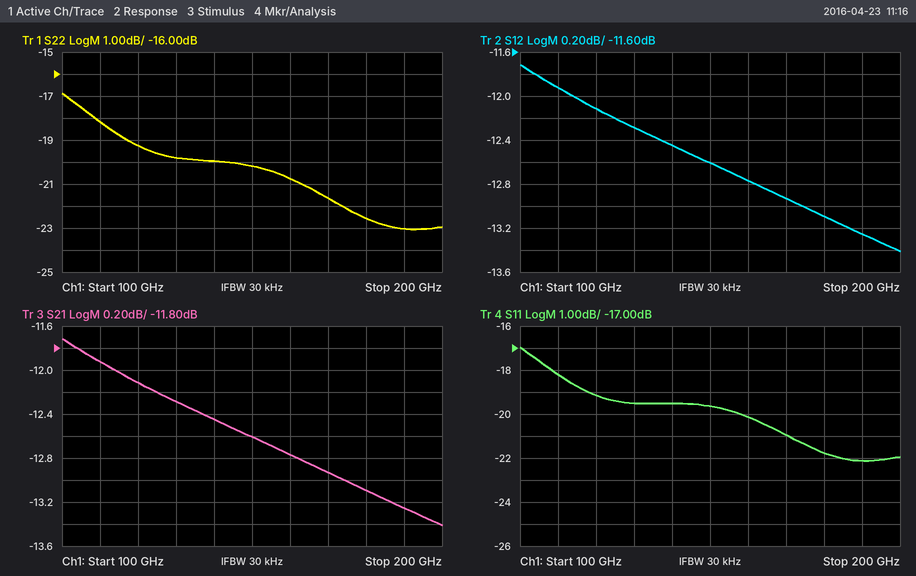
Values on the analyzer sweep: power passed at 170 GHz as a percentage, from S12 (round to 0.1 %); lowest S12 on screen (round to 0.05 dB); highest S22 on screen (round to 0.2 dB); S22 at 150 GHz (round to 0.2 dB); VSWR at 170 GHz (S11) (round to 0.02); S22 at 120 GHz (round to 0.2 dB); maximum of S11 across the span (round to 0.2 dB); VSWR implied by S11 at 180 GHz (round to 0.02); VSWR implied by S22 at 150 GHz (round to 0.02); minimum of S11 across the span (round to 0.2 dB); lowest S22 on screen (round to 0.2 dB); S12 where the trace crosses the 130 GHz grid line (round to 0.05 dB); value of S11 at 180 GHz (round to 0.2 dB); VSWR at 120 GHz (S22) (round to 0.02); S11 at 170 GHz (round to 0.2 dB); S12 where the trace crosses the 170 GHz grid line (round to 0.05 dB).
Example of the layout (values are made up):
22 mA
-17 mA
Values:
5.1 %
-13.40 dB
-16.8 dB
-20.2 dB
1.20
-19.2 dB
-17.0 dB
1.18
1.22
-22.2 dB
-23.0 dB
-12.30 dB
-21.8 dB
1.24
-21.0 dB
-12.95 dB
